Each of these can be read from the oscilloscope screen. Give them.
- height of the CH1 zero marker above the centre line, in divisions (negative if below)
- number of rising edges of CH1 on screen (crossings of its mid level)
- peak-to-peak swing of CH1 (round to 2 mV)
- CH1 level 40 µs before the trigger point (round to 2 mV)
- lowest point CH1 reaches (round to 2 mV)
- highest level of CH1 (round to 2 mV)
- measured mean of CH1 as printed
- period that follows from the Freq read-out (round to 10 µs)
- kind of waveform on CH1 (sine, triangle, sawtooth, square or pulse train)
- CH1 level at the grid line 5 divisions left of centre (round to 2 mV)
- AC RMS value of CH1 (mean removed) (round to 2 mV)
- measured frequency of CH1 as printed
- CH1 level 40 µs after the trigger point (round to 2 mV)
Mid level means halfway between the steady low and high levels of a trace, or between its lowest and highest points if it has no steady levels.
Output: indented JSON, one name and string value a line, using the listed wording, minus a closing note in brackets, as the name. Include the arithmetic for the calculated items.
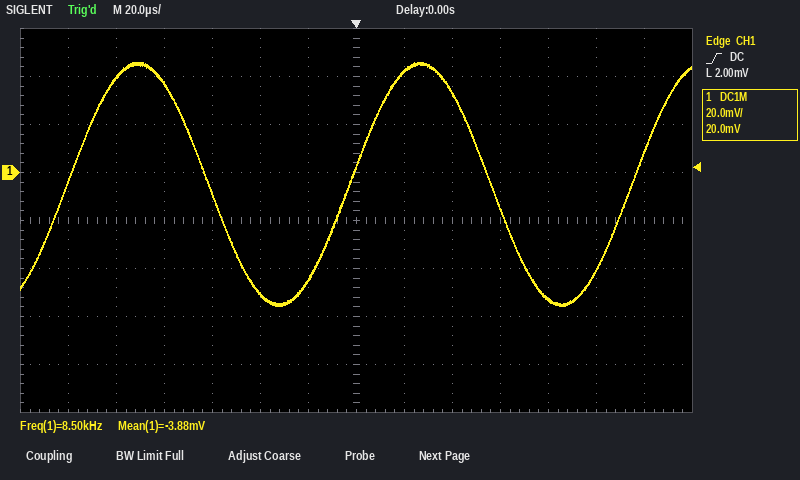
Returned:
{
  "height of the CH1 zero marker above the centre line, in divisions": "+1.0 div",
  "number of rising edges of CH1 on screen": "3",
  "peak-to-peak swing of CH1": "46 mV − (-56 mV) = 102 mV",
  "CH1 level 40 µs before the trigger point": "-50 mV",
  "lowest point CH1 reaches": "-56 mV",
  "highest level of CH1": "46 mV",
  "measured mean of CH1 as printed": "-3.88 mV",
  "period that follows from the Freq read-out": "1 / 8.50 kHz ≈ 118 µs, so 120 µs to the nearest 10 µs",
  "kind of waveform on CH1": "sine",
  "CH1 level at the grid line 5 divisions left of centre": "40 mV",
  "AC RMS value of CH1 (mean removed)": "102 mV / (2√2) ≈ 36 mV",
  "measured frequency of CH1 as printed": "8.50 kHz",
  "CH1 level 40 µs after the trigger point": "34 mV"
}
